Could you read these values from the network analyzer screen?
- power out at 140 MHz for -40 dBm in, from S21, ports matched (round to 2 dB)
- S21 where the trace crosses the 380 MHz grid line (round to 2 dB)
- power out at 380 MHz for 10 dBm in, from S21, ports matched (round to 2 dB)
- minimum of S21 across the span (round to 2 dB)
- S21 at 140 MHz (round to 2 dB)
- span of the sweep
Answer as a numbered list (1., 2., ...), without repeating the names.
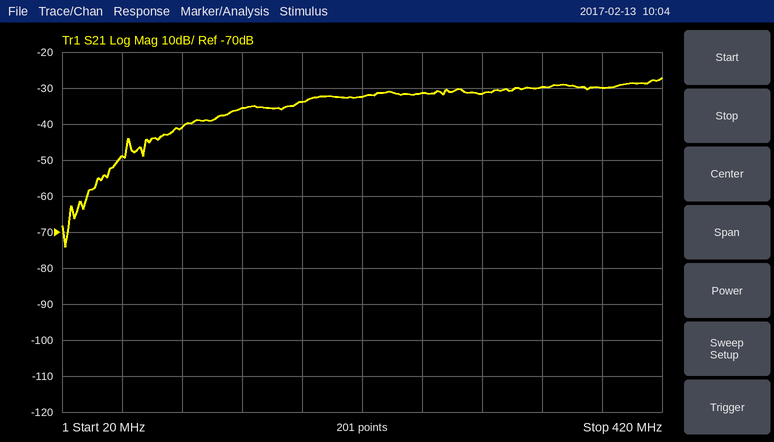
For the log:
1. -76 dBm
2. -30 dB
3. -20 dBm
4. -74 dB
5. -36 dB
6. 400 MHz
